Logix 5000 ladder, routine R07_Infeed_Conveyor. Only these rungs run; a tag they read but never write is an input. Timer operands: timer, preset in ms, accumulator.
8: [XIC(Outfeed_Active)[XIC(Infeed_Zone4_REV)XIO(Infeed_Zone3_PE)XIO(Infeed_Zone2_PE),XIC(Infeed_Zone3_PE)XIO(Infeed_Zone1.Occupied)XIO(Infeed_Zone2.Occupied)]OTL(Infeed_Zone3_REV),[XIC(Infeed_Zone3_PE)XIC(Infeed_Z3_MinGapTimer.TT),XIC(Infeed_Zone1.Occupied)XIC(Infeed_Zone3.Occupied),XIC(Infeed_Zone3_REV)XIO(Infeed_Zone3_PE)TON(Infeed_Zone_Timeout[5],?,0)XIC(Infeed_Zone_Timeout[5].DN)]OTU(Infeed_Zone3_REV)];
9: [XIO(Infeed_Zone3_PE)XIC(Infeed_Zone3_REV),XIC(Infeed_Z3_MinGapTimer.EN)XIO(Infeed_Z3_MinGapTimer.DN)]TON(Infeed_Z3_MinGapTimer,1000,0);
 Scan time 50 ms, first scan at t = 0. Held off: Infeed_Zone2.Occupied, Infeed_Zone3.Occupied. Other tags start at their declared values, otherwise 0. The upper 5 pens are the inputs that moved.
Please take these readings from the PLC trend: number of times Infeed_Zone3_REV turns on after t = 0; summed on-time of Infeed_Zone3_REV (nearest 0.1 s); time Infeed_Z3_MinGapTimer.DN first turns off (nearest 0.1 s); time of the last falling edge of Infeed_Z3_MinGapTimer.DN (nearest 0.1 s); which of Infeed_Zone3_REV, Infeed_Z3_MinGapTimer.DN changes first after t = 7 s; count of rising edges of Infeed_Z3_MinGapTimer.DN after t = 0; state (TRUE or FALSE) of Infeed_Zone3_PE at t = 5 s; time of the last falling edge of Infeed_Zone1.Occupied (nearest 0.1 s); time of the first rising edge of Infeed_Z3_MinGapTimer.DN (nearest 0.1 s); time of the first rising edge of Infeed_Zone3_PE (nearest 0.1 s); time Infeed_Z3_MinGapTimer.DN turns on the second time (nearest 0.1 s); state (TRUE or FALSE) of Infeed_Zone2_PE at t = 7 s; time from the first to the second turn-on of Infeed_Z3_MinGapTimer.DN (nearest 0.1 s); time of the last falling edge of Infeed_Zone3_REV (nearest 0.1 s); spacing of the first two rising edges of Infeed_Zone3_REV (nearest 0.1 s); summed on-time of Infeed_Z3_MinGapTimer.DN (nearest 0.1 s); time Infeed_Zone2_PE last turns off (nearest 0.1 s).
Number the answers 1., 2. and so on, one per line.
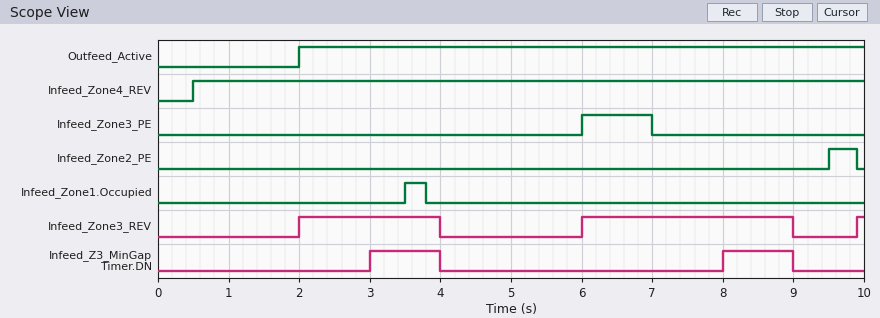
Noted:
1. 3
2. 5.1 s
3. 4.0 s
4. 9.0 s
5. Infeed_Z3_MinGapTimer.DN
6. 2
7. FALSE
8. 3.8 s
9. 3.0 s
10. 6.0 s
11. 8.0 s
12. FALSE
13. 5.0 s
14. 9.0 s
15. 4.0 s
16. 2.0 s
17. 9.9 s
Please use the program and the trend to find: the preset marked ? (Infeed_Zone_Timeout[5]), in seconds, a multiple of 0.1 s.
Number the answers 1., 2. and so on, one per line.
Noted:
1. 2.0 s
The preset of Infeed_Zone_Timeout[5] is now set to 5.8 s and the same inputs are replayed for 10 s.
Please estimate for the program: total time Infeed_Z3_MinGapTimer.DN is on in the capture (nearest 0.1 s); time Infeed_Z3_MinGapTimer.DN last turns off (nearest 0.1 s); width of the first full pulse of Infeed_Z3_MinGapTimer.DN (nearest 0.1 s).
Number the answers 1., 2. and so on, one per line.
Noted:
1. 5.0 s
2. 6.0 s
3. 3.0 s
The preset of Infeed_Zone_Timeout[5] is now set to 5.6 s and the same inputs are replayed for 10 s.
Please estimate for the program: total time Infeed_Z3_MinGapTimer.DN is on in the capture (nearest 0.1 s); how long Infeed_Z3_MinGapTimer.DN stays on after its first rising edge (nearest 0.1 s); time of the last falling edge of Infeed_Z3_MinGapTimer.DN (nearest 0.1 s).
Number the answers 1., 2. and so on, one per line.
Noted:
1. 5.0 s
2. 3.0 s
3. 6.0 s
